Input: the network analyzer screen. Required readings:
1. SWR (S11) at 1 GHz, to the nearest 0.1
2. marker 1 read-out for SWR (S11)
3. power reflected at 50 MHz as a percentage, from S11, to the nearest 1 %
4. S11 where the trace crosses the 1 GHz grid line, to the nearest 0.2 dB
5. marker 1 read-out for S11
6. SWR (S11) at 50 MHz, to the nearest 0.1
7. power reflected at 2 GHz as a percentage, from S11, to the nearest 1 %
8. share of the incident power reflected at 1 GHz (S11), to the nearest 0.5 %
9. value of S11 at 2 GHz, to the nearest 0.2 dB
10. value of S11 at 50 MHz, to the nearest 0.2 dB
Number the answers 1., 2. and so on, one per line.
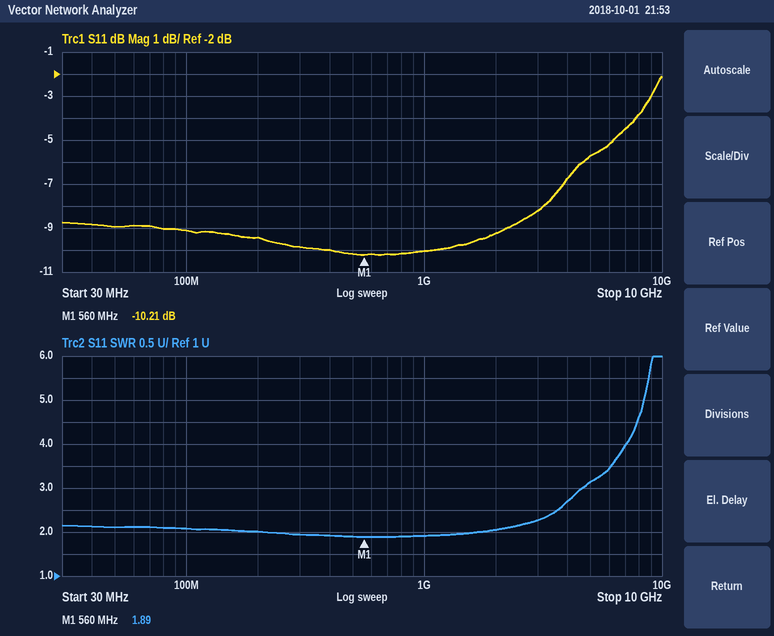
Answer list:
1. 1.9
2. 1.89
3. 13 %
4. -10.0 dB
5. -10.21 dB
6. 2.1
7. 12 %
8. 10.0 %
9. -9.2 dB
10. -9.0 dB
